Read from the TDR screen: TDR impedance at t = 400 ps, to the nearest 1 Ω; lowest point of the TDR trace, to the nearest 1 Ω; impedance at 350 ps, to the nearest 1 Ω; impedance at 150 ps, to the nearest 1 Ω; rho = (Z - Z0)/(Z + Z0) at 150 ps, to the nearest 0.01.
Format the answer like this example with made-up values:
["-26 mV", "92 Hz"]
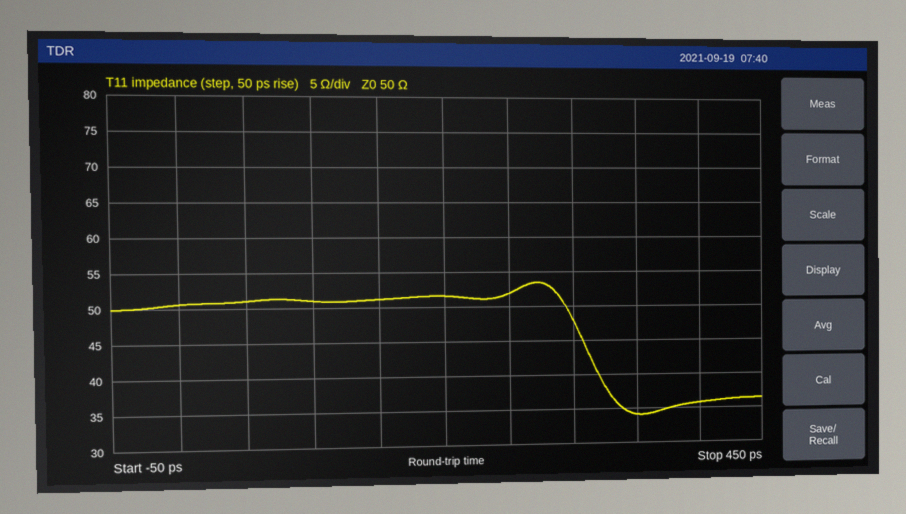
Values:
["36 Ω", "34 Ω", "34 Ω", "51 Ω", "+0.01"]
